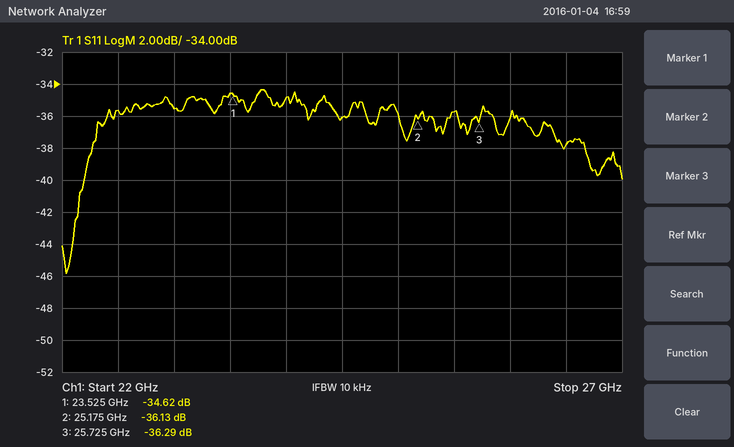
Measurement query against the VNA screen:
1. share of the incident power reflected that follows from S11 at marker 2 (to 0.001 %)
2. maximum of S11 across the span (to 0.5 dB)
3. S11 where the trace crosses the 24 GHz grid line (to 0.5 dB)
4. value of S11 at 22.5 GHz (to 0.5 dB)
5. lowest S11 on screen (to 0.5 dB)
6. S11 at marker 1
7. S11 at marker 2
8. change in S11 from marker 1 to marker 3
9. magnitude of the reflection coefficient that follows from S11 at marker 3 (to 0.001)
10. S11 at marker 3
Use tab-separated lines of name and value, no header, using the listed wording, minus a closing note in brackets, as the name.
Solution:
share of the incident power reflected that follows from S11 at marker 2	0.024 %
maximum of S11 across the span	-34.5 dB
S11 where the trace crosses the 24 GHz grid line	-35.0 dB
value of S11 at 22.5 GHz	-35.5 dB
lowest S11 on screen	-46.0 dB
S11 at marker 1	-34.62 dB
S11 at marker 2	-36.13 dB
change in S11 from marker 1 to marker 3	-1.67 dB
magnitude of the reflection coefficient that follows from S11 at marker 3	0.015
S11 at marker 3	-36.29 dB
